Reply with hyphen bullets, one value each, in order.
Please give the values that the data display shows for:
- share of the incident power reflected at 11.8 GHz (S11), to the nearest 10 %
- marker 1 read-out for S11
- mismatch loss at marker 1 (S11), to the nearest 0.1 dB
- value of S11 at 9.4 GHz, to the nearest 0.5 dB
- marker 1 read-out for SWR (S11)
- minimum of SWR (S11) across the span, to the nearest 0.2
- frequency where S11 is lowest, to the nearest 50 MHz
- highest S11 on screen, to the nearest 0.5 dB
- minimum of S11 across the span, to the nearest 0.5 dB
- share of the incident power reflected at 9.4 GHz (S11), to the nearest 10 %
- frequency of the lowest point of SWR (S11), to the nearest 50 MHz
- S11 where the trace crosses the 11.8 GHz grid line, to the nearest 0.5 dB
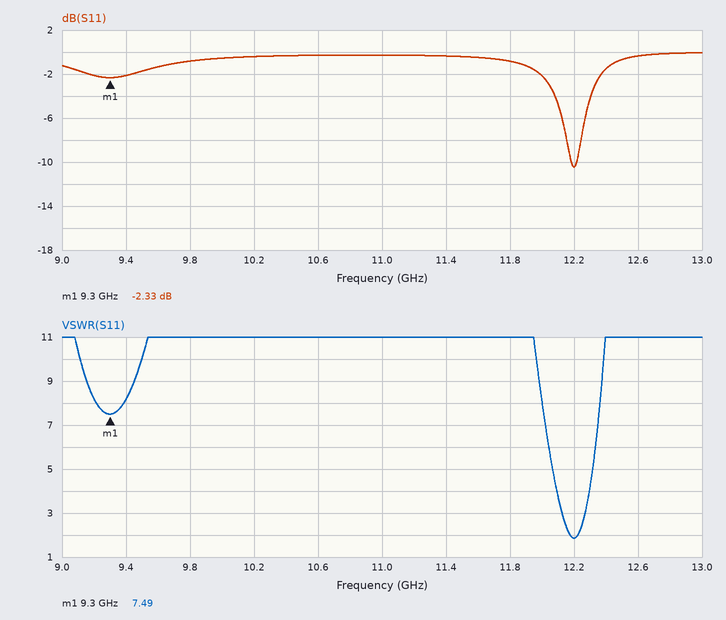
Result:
- 80 %
- -2.33 dB
- 3.8 dB
- -2.0 dB
- 7.49
- 1.8
- 12.20 GHz
- 0.0 dB
- -10.5 dB
- 60 %
- 12.20 GHz
- -1.0 dB
